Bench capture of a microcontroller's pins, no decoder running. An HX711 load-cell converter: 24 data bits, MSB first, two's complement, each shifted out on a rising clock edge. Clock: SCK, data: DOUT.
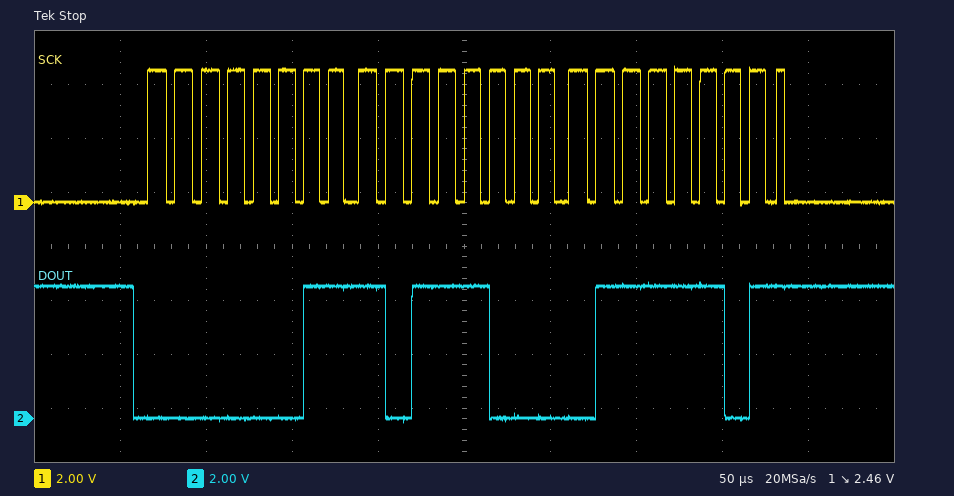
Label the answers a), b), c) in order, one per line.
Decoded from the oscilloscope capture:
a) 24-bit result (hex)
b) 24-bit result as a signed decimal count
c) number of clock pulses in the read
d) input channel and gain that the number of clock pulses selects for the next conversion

a) 0x03B87D
b) 243837
c) 25
d) channel A, gain 128
